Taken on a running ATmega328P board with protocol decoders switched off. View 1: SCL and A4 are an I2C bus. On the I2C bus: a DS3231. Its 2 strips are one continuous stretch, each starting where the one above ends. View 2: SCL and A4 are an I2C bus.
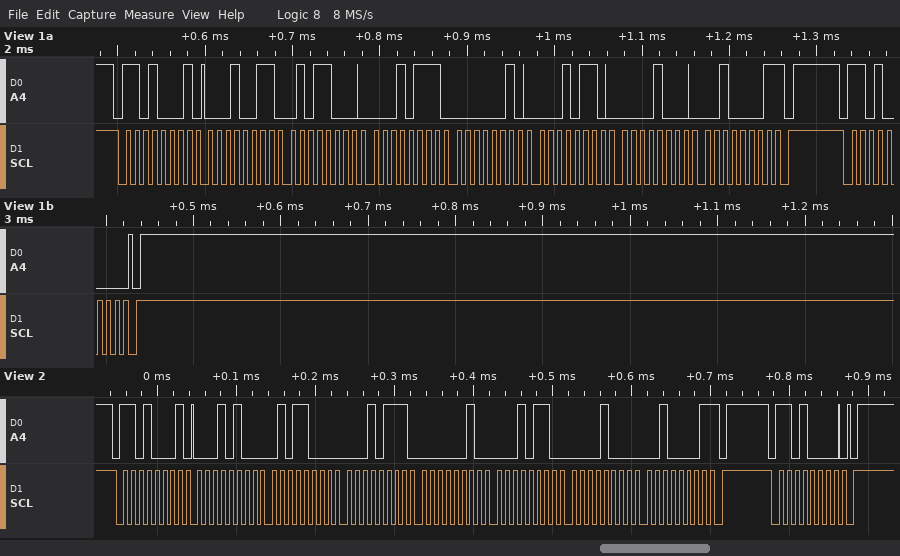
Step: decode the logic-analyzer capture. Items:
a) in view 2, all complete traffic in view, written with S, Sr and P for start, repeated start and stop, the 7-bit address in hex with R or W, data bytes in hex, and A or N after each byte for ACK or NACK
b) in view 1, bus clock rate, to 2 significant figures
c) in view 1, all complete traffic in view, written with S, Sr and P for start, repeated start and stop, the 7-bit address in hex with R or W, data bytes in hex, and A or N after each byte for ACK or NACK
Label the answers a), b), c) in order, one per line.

a) S 68R A 14 A 58 A 17 A 02 A 16 A 08 A 21 N P S 68W A P
b) 100 kHz
c) S 68R A 13 A 58 A 17 A 02 A 16 A 08 A 21 N P S 68W A P
